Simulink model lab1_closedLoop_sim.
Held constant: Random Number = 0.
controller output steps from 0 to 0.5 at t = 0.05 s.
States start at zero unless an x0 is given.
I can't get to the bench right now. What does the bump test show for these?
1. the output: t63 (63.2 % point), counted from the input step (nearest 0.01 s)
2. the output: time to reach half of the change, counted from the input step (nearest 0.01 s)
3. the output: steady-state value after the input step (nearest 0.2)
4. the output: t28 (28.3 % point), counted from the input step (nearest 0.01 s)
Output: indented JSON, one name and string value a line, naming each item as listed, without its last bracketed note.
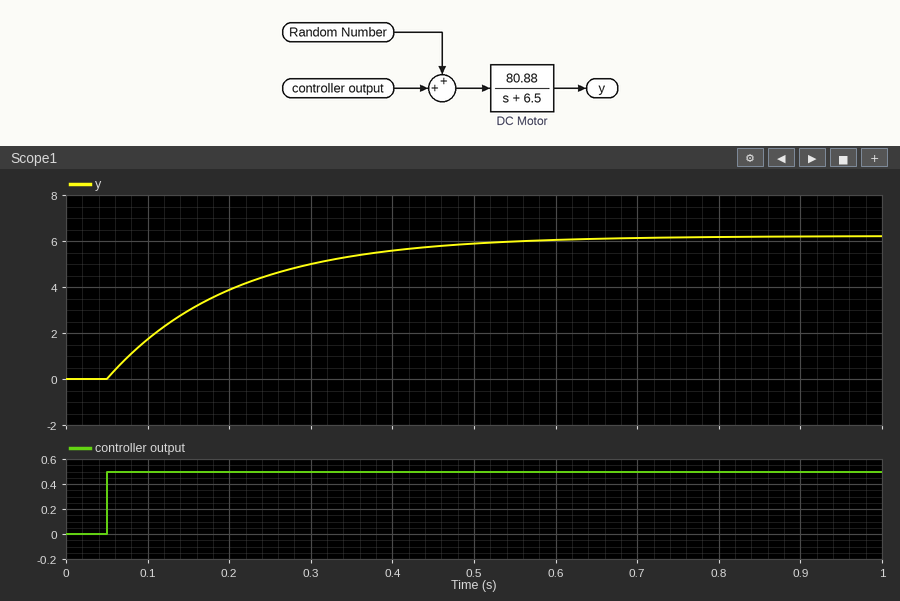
{
  "the output: t63 (63.2 % point), counted from the input step": "0.15 s",
  "the output: time to reach half of the change, counted from the input step": "0.11 s",
  "the output: steady-state value after the input step": "6.2",
  "the output: t28 (28.3 % point), counted from the input step": "0.05 s"
}
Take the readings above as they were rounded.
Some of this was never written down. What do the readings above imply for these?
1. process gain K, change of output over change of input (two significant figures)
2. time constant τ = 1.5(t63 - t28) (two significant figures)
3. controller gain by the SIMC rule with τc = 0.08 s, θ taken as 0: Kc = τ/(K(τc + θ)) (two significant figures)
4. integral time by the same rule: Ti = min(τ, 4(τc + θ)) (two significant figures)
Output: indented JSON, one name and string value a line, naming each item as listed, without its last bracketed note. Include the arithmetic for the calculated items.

{
  "process gain K, change of output over change of input": "(6.2 - 0) / 0.5 = 12",
  "time constant τ = 1.5(t63 - t28)": "1.5 × (0.15 - 0.05) = 0.15 s",
  "controller gain by the SIMC rule with τc = 0.08 s, θ taken as 0: Kc = τ/(K(τc + θ))": "0.15 / (12 × (0.08 + 0)) = 0.16",
  "integral time by the same rule: Ti = min(τ, 4(τc + θ))": "min(0.15, 4 × (0.08 + 0)) = 0.15 s"
}
